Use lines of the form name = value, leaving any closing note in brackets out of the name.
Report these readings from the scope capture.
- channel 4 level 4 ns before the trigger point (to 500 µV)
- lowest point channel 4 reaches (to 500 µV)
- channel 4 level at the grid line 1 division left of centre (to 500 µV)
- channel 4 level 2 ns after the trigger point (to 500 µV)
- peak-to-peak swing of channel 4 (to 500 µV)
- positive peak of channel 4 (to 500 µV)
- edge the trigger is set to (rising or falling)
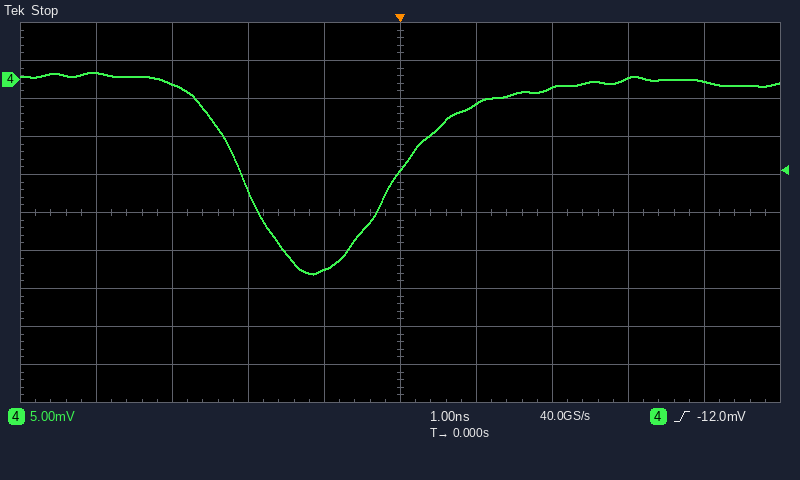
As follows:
channel 4 level 4 ns before the trigger point = 1.0 mV
lowest point channel 4 reaches = -25.5 mV
channel 4 level at the grid line 1 division left of centre = -25.0 mV
channel 4 level 2 ns after the trigger point = -1.0 mV
peak-to-peak swing of channel 4 = 26.5 mV
positive peak of channel 4 = 1.0 mV
edge the trigger is set to = rising
